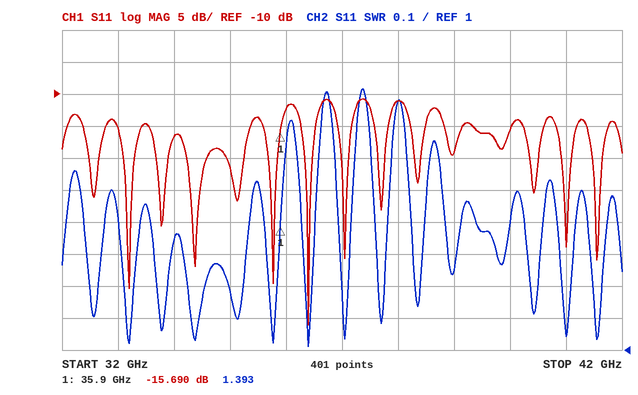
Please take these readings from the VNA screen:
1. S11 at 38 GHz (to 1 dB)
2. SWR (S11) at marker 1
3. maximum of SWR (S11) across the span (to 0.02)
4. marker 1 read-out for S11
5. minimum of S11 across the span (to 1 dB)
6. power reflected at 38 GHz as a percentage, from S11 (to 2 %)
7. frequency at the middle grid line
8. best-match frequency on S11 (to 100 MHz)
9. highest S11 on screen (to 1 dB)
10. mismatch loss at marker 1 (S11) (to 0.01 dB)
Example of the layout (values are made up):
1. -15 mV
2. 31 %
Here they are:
1. -11 dB
2. 1.393
3. 1.82
4. -15.690 dB
5. -46 dB
6. 8 %
7. 37 GHz
8. 36.4 GHz
9. -11 dB
10. 0.12 dB
